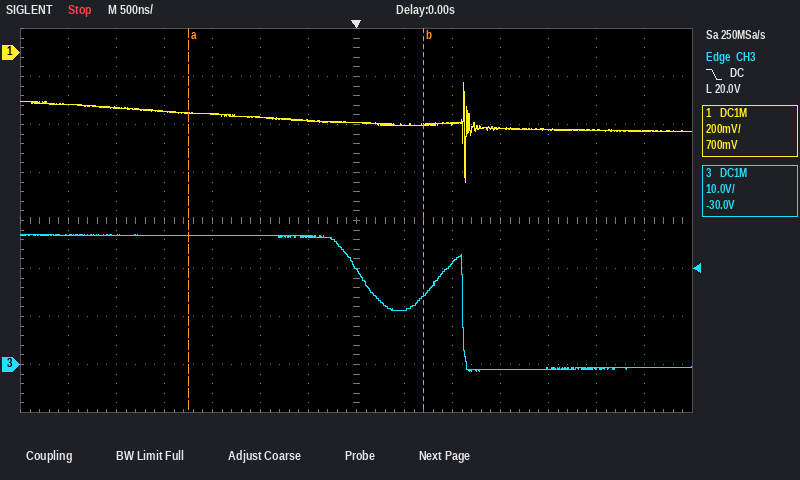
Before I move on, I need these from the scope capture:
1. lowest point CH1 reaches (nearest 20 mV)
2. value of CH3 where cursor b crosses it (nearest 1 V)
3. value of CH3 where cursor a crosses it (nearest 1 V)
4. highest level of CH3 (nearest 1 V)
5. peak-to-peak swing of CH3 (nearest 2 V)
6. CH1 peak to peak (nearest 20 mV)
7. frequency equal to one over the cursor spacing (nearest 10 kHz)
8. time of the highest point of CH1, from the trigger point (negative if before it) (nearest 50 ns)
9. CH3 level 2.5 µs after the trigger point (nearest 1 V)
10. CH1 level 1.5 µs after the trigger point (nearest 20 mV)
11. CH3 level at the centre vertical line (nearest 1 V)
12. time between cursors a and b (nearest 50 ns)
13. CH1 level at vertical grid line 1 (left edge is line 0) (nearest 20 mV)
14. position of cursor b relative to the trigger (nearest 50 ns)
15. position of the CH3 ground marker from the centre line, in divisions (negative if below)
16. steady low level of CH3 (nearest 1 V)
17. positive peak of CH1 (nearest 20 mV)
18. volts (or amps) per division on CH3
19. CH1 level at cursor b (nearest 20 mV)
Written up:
-540 mV
14 V
27 V
27 V
28 V
420 mV
410 kHz
+1.10 µs
-1 V
-320 mV
20 V
2.45 µs
-220 mV
+700 ns
-3.0 div
-1 V
-120 mV
10 V
-300 mV
